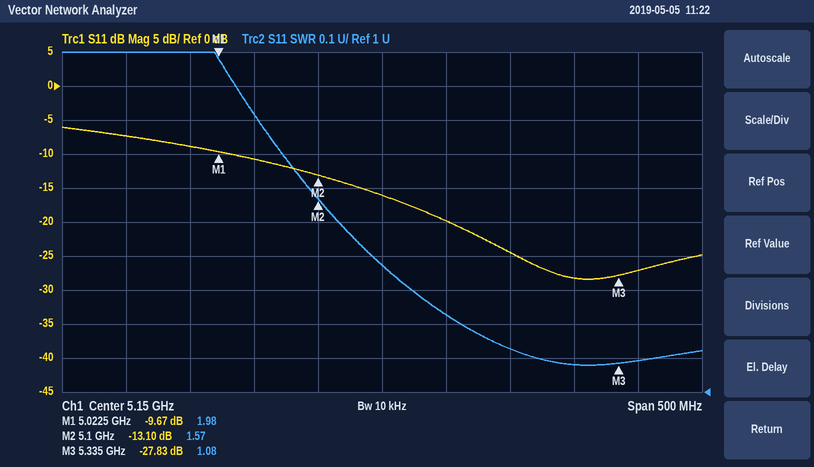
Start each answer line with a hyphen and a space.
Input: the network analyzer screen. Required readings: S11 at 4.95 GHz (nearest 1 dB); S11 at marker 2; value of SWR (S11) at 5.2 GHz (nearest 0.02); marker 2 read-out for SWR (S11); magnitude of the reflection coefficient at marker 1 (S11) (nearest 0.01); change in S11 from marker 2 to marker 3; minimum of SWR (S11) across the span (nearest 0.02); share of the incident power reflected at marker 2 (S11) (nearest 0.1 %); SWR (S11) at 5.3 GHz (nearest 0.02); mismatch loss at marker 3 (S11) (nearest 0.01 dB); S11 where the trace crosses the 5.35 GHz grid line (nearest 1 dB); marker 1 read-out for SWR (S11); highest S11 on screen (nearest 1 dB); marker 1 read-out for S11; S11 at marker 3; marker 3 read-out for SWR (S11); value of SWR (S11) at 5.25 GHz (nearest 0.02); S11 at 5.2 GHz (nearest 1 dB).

- -7 dB
- -13.10 dB
- 1.22
- 1.57
- 0.33
- -14.73 dB
- 1.08
- 4.9 %
- 1.08
- 0.01 dB
- -27 dB
- 1.98
- -6 dB
- -9.67 dB
- -27.83 dB
- 1.08
- 1.12
- -20 dB
